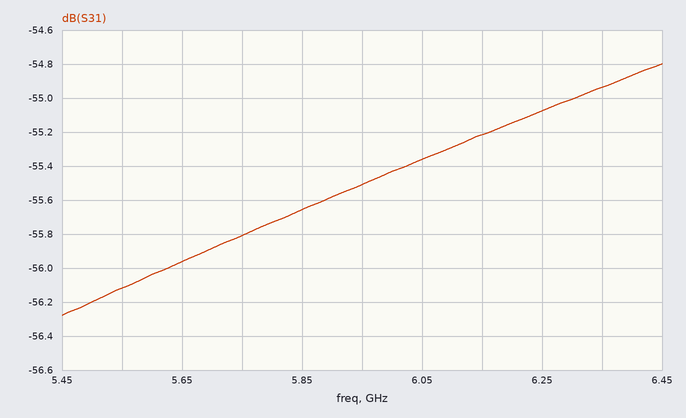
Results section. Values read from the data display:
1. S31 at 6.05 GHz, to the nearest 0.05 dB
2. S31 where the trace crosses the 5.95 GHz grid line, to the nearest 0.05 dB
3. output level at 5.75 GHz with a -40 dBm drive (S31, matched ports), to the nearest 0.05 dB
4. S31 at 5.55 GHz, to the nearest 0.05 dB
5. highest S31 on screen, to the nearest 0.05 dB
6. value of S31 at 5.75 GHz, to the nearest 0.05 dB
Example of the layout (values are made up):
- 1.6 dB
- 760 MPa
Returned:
- -55.35 dB
- -55.50 dB
- -95.80 dBm
- -56.10 dB
- -54.80 dB
- -55.80 dB
